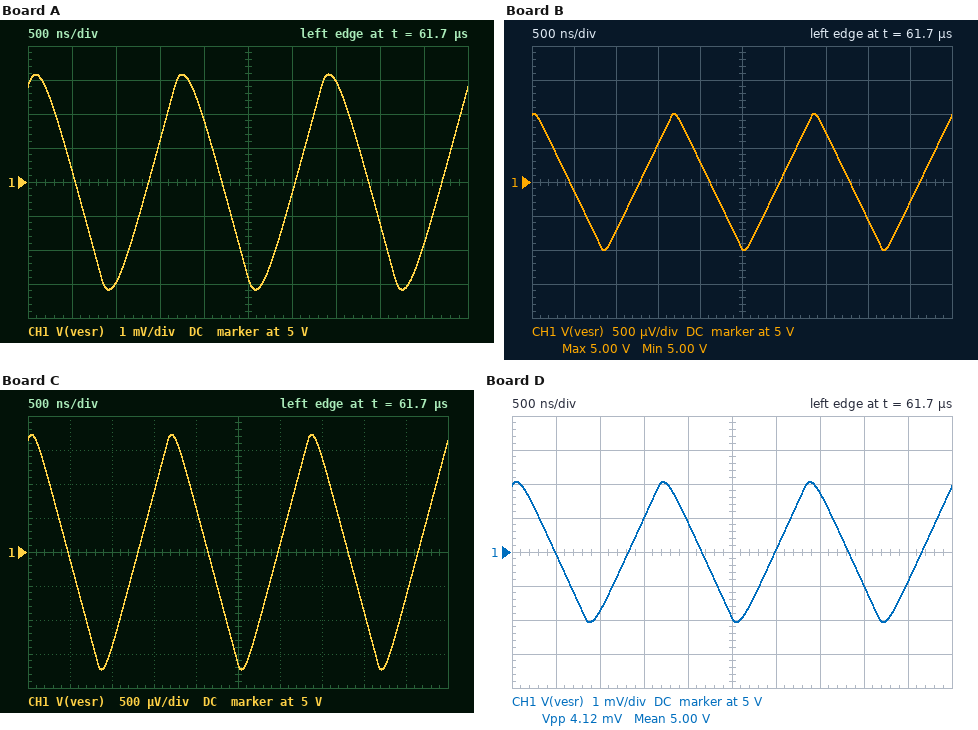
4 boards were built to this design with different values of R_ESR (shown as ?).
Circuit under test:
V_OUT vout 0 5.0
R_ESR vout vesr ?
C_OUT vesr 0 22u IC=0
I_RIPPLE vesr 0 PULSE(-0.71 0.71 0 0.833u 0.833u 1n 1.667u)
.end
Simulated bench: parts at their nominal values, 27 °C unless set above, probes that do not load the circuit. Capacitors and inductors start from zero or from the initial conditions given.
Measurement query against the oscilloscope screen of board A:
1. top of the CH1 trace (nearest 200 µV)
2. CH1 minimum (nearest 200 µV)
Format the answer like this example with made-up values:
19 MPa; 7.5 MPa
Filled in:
5.0032 V; 4.9968 V
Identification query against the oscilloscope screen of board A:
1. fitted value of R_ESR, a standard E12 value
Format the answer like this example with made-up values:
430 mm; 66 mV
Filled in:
5.6 mΩ
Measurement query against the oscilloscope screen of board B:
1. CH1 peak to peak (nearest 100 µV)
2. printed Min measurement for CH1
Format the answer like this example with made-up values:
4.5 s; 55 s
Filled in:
2.0 mV; 5.00 V
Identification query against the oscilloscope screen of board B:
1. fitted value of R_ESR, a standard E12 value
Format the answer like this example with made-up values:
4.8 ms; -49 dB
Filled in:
1.5 mΩ
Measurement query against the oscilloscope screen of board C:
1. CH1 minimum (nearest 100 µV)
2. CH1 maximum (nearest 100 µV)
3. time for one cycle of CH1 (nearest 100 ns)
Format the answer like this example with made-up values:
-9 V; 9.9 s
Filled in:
4.9983 V; 5.0017 V; 1.7 µs
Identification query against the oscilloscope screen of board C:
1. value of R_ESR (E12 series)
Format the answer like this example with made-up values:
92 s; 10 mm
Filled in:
2.7 mΩ
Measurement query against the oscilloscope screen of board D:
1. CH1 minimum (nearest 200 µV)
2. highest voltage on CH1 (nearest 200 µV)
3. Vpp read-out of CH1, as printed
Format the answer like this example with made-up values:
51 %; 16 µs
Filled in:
4.9980 V; 5.0020 V; 4.12 mV
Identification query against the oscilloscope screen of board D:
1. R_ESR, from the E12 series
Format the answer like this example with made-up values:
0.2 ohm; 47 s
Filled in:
3.3 mΩ
